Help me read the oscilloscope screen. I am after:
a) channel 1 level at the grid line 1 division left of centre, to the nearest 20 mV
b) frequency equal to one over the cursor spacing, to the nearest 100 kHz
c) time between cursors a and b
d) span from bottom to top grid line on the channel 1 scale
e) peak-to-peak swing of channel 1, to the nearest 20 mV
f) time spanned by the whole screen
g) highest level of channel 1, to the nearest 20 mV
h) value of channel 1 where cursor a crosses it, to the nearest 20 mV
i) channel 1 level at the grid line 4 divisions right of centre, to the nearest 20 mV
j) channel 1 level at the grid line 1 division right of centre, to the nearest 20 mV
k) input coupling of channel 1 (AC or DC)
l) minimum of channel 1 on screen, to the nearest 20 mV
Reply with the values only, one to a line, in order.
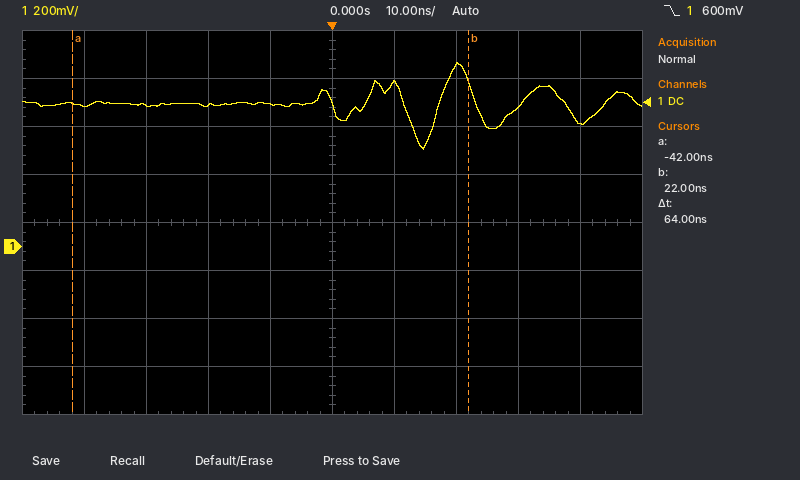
600 mV
15.6 MHz
64 ns
1.6 V
360 mV
100 ns
760 mV
600 mV
520 mV
680 mV
DC
400 mV
